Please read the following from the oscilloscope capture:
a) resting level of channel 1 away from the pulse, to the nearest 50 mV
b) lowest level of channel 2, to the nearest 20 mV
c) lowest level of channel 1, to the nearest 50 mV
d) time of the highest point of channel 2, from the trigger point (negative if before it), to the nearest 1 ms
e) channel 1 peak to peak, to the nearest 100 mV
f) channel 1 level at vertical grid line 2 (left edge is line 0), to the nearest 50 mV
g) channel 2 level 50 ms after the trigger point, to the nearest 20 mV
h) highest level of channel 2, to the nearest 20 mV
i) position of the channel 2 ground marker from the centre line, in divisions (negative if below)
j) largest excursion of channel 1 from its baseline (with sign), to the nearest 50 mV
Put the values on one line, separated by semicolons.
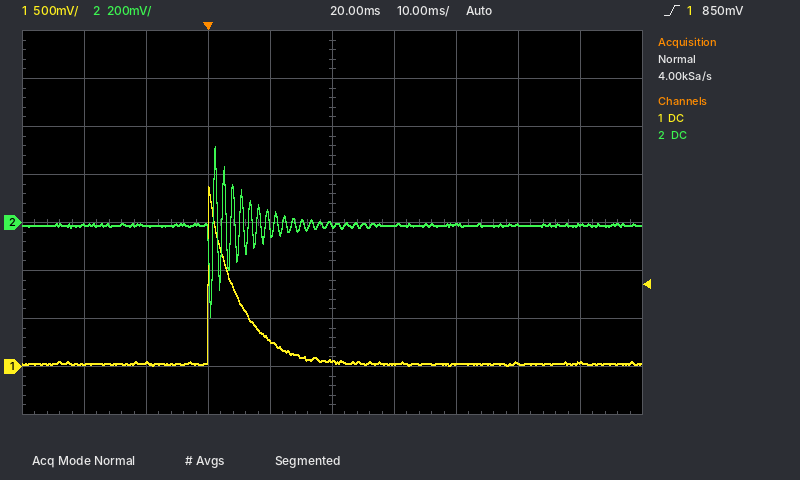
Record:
50 mV; -400 mV; 0 mV; +1 ms; 1.90 V; 50 mV; 0 mV; 320 mV; 0.0 div; +1.85 V
